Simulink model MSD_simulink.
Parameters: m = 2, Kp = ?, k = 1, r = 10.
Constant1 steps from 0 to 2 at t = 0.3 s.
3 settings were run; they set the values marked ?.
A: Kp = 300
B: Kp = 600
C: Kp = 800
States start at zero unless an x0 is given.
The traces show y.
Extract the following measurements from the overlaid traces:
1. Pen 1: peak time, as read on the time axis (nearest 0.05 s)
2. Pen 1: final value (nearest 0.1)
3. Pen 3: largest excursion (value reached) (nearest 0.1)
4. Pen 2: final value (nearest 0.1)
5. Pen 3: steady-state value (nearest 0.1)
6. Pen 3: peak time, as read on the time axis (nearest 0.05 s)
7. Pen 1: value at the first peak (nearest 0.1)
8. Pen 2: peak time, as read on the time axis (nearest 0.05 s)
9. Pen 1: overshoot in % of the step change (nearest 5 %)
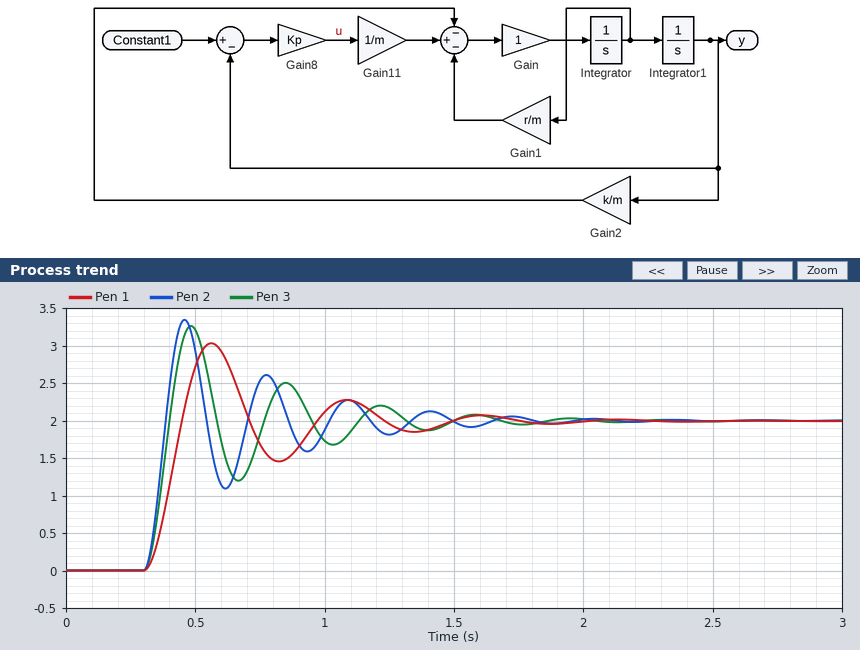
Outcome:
0.55 s
2.0
3.3
2.0
2.0
0.50 s
3.0
0.45 s
50 %
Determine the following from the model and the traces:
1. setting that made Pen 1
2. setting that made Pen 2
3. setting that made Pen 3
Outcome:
A
C
B
